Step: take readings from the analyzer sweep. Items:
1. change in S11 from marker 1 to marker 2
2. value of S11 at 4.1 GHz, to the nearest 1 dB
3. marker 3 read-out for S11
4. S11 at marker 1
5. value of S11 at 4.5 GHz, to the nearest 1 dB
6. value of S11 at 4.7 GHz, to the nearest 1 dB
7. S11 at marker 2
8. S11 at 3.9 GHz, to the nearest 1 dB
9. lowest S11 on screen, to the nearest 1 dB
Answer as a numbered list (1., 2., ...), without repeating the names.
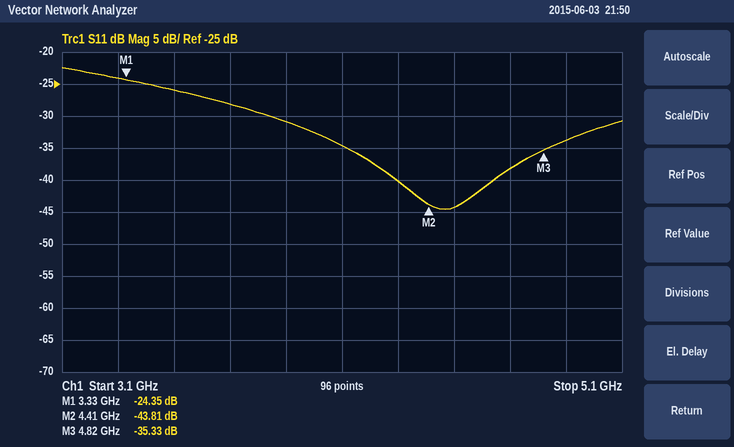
1. -19.46 dB
2. -35 dB
3. -35.33 dB
4. -24.35 dB
5. -44 dB
6. -38 dB
7. -43.81 dB
8. -31 dB
9. -45 dB
